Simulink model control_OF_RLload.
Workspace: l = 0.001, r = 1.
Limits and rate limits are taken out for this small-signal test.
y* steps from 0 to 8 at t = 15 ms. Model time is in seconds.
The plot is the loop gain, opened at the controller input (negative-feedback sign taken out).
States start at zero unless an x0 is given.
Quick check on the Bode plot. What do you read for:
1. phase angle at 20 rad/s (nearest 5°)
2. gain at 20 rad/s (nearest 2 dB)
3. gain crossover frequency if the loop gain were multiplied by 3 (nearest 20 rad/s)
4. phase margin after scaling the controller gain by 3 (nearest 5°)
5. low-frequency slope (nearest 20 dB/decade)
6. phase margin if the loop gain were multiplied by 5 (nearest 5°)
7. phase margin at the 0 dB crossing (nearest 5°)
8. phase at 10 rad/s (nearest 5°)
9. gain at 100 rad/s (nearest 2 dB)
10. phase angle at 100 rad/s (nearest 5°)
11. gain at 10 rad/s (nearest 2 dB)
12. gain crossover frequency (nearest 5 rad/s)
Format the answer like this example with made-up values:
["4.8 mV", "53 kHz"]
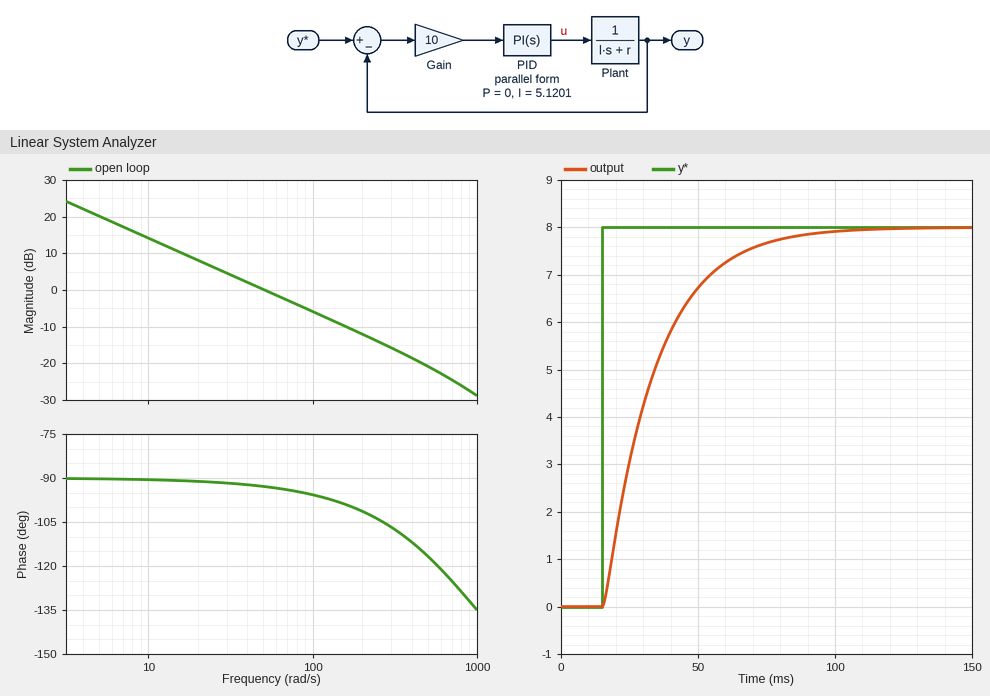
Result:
["-90°", "8 dB", "160 rad/s", "80°", "-20 dB/decade", "75°", "85°", "-90°", "-6 dB", "-95°", "14 dB", "50 rad/s"]
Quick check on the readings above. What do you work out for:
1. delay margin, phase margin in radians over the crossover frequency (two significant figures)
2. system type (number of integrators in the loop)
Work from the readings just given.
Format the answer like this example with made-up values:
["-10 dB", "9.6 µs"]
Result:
["0.030 s", "1"]
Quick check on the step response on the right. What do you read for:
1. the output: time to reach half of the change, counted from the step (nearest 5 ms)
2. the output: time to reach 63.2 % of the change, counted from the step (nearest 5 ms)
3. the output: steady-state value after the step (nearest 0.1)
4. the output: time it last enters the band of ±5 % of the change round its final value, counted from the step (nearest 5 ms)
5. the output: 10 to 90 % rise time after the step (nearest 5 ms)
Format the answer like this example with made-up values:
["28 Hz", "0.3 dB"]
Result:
["15 ms", "20 ms", "8.0", "55 ms", "40 ms"]
